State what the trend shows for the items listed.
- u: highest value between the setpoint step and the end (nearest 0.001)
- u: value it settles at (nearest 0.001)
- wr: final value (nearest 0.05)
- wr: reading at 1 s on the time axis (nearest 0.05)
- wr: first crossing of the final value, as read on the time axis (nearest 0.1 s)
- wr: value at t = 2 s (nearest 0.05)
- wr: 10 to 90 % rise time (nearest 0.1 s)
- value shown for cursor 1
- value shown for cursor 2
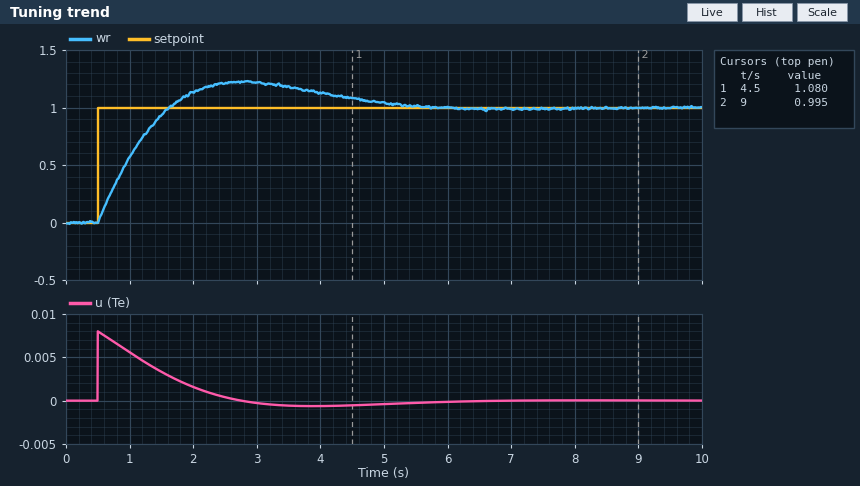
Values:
0.008
0.000
1.00
0.55
1.6 s
1.15
0.9 s
1.080
0.995
